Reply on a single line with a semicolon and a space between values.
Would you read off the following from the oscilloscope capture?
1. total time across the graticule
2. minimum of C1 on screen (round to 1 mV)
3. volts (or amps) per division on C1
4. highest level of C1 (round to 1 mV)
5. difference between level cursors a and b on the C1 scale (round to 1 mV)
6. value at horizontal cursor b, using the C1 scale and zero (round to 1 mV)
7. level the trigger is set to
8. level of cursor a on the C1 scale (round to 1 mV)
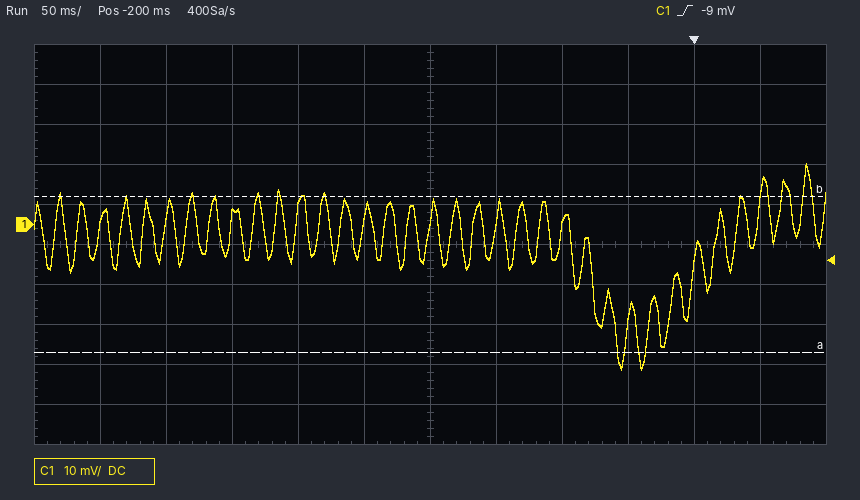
600 ms; -36 mV; 10 mV; 15 mV; 39 mV; 7 mV; -9 mV; -32 mV
